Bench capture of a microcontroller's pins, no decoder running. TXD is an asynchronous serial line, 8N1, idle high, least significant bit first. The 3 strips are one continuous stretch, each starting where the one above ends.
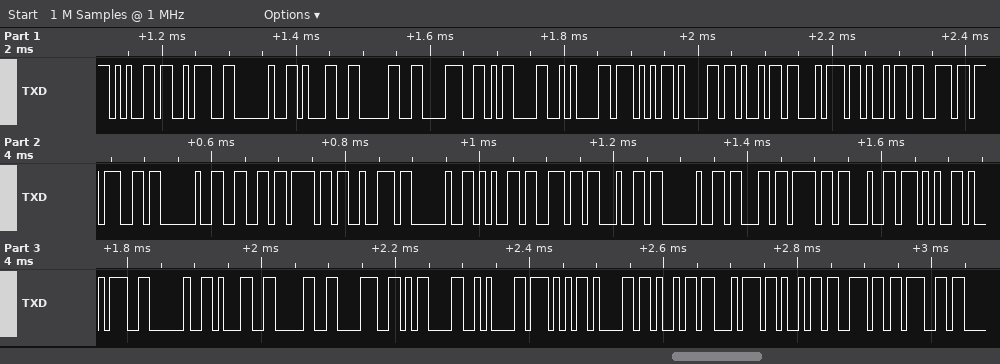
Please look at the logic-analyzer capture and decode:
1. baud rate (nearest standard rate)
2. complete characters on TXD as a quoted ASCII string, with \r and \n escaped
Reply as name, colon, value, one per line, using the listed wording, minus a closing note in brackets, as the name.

baud rate: 115200 baud
complete characters on TXD as a quoted ASCII string, with \r and \n escaped: "e: 108\r\nWaiting for end code: 108\r\nWaiting"
